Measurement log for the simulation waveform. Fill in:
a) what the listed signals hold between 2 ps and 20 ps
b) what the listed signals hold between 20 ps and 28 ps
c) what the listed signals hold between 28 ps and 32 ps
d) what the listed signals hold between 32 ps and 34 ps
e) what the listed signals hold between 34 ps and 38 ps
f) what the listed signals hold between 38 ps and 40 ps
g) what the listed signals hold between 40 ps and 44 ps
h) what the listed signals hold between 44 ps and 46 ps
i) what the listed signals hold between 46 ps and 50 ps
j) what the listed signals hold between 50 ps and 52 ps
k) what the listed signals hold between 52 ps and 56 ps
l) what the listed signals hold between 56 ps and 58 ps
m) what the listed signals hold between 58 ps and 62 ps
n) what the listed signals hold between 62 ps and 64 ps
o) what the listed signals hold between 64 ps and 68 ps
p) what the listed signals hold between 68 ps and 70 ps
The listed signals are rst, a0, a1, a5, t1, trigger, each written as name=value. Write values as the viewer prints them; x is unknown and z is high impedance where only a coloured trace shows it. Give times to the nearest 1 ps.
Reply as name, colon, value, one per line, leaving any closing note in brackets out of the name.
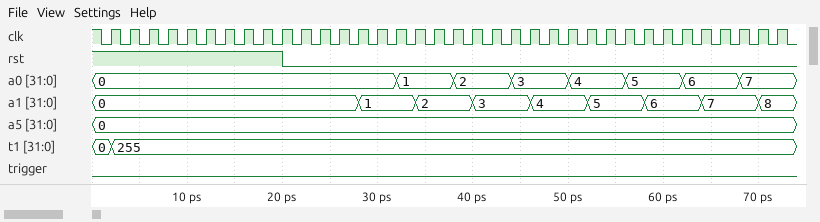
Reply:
what the listed signals hold between 2 ps and 20 ps: rst=1, a0=0, a1=0, a5=0, t1=255, trigger=0
what the listed signals hold between 20 ps and 28 ps: rst=0, a0=0, a1=0, a5=0, t1=255, trigger=0
what the listed signals hold between 28 ps and 32 ps: rst=0, a0=0, a1=1, a5=0, t1=255, trigger=0
what the listed signals hold between 32 ps and 34 ps: rst=0, a0=1, a1=1, a5=0, t1=255, trigger=0
what the listed signals hold between 34 ps and 38 ps: rst=0, a0=1, a1=2, a5=0, t1=255, trigger=0
what the listed signals hold between 38 ps and 40 ps: rst=0, a0=2, a1=2, a5=0, t1=255, trigger=0
what the listed signals hold between 40 ps and 44 ps: rst=0, a0=2, a1=3, a5=0, t1=255, trigger=0
what the listed signals hold between 44 ps and 46 ps: rst=0, a0=3, a1=3, a5=0, t1=255, trigger=0
what the listed signals hold between 46 ps and 50 ps: rst=0, a0=3, a1=4, a5=0, t1=255, trigger=0
what the listed signals hold between 50 ps and 52 ps: rst=0, a0=4, a1=4, a5=0, t1=255, trigger=0
what the listed signals hold between 52 ps and 56 ps: rst=0, a0=4, a1=5, a5=0, t1=255, trigger=0
what the listed signals hold between 56 ps and 58 ps: rst=0, a0=5, a1=5, a5=0, t1=255, trigger=0
what the listed signals hold between 58 ps and 62 ps: rst=0, a0=5, a1=6, a5=0, t1=255, trigger=0
what the listed signals hold between 62 ps and 64 ps: rst=0, a0=6, a1=6, a5=0, t1=255, trigger=0
what the listed signals hold between 64 ps and 68 ps: rst=0, a0=6, a1=7, a5=0, t1=255, trigger=0
what the listed signals hold between 68 ps and 70 ps: rst=0, a0=7, a1=7, a5=0, t1=255, trigger=0
